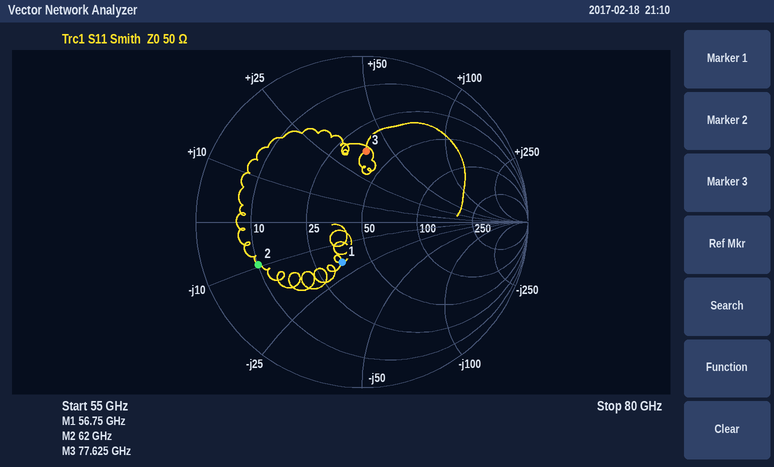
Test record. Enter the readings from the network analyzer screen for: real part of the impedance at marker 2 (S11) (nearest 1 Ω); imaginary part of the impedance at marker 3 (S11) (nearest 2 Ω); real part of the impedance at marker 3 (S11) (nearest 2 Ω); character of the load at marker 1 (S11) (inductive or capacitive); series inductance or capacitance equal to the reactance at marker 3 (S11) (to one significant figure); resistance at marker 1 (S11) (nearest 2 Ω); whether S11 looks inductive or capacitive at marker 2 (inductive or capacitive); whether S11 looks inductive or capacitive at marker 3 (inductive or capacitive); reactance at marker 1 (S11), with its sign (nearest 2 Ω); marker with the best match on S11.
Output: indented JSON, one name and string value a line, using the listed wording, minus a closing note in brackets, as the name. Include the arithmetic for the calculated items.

{
  "real part of the impedance at marker 2 (S11)": "10 Ω",
  "imaginary part of the impedance at marker 3 (S11)": "+38 Ω",
  "real part of the impedance at marker 3 (S11)": "36 Ω",
  "character of the load at marker 1 (S11)": "capacitive",
  "series inductance or capacitance equal to the reactance at marker 3 (S11)": "L = 38 Ω/(2π × 77.625 GHz) ≈ 77.9 pH, so 80 pH to one significant figure",
  "resistance at marker 1 (S11)": "36 Ω",
  "whether S11 looks inductive or capacitive at marker 2": "capacitive",
  "whether S11 looks inductive or capacitive at marker 3": "inductive",
  "reactance at marker 1 (S11), with its sign": "-18 Ω",
  "marker with the best match on S11": "marker 1"
}
